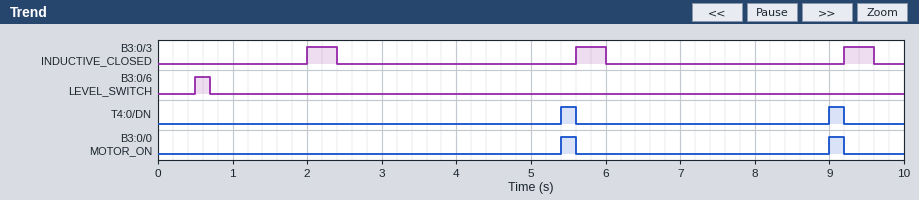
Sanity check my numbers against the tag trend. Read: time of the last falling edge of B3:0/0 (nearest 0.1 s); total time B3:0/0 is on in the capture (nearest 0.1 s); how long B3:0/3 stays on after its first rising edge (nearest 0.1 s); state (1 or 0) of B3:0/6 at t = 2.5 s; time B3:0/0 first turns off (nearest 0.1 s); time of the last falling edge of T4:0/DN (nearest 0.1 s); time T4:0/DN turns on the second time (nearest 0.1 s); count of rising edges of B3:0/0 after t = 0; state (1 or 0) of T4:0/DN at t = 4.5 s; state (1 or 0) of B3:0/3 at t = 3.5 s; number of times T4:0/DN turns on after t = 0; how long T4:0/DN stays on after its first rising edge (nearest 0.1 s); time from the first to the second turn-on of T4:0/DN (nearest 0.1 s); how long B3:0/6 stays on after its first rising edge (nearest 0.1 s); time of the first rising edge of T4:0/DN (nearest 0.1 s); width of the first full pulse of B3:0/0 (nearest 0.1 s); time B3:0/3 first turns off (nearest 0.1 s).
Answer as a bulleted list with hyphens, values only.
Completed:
- 9.2 s
- 0.4 s
- 0.4 s
- 0
- 5.6 s
- 9.2 s
- 9.0 s
- 2
- 0
- 0
- 2
- 0.2 s
- 3.6 s
- 0.2 s
- 5.4 s
- 0.2 s
- 2.4 s
